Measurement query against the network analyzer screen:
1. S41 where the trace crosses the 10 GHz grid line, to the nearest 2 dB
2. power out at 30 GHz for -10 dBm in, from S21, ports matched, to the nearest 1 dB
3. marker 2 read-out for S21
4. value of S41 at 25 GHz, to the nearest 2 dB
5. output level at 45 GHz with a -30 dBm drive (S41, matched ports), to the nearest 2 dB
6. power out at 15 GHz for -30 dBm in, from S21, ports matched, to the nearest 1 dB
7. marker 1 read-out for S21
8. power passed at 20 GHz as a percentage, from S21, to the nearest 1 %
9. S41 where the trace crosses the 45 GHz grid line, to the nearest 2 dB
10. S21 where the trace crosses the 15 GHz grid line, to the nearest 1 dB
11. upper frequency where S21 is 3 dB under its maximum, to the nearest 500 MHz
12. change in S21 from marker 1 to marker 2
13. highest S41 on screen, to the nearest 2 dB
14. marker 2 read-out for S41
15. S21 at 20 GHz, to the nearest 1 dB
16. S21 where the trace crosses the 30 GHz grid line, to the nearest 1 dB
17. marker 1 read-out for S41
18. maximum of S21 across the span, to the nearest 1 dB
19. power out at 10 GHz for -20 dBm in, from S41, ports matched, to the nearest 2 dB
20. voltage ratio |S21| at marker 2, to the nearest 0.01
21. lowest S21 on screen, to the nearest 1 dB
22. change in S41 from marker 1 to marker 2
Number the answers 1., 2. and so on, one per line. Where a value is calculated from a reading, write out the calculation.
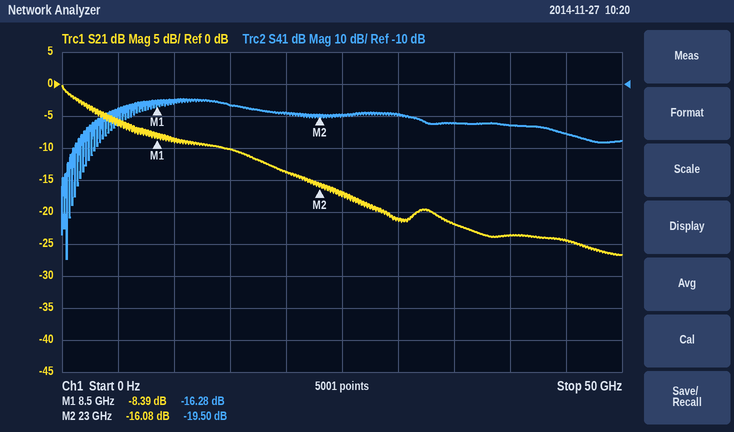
1. -16 dB
2. -10 dBm + (-21 dB) = -31 dBm
3. -16.08 dB
4. -20 dB
5. -30 dBm + (-26 dB) = -56 dBm
6. -30 dBm + (-10 dB) = -40 dBm
7. -8.39 dB
8. 10^(-14/10) ≈ 4 %
9. -26 dB
10. -10 dB
11. 2.0 GHz
12. -16.08 − (-8.39) = -7.69 dB
13. -14 dB
14. -19.50 dB
15. -14 dB
16. -21 dB
17. -16.28 dB
18. 0 dB
19. -20 dBm + (-16 dB) = -36 dBm
20. 10^(-16.08/20) ≈ 0.16
21. -27 dB
22. -19.5 − (-16.28) = -3.22 dB
